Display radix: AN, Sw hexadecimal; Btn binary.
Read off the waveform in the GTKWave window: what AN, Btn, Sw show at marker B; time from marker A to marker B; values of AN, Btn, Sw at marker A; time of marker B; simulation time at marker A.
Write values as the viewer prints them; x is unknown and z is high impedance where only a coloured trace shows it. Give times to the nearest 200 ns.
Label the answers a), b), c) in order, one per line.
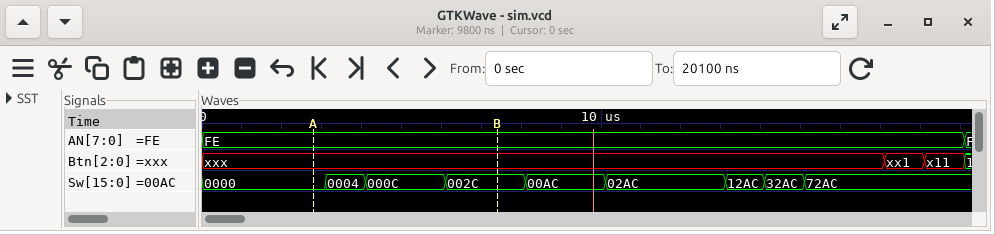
a) AN=FE, Btn=xxx, Sw=002C
b) 4600 ns
c) AN=FE, Btn=xxx, Sw=0000
d) 7400 ns
e) 2800 ns
